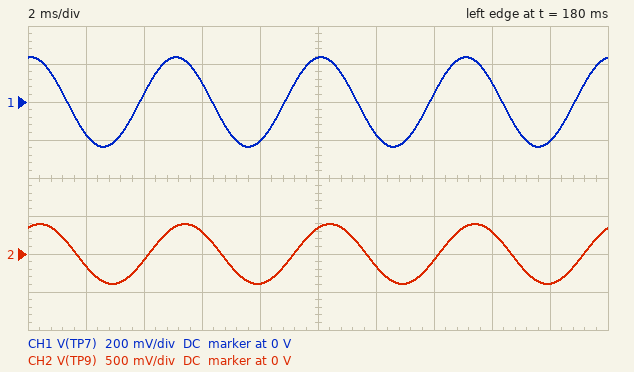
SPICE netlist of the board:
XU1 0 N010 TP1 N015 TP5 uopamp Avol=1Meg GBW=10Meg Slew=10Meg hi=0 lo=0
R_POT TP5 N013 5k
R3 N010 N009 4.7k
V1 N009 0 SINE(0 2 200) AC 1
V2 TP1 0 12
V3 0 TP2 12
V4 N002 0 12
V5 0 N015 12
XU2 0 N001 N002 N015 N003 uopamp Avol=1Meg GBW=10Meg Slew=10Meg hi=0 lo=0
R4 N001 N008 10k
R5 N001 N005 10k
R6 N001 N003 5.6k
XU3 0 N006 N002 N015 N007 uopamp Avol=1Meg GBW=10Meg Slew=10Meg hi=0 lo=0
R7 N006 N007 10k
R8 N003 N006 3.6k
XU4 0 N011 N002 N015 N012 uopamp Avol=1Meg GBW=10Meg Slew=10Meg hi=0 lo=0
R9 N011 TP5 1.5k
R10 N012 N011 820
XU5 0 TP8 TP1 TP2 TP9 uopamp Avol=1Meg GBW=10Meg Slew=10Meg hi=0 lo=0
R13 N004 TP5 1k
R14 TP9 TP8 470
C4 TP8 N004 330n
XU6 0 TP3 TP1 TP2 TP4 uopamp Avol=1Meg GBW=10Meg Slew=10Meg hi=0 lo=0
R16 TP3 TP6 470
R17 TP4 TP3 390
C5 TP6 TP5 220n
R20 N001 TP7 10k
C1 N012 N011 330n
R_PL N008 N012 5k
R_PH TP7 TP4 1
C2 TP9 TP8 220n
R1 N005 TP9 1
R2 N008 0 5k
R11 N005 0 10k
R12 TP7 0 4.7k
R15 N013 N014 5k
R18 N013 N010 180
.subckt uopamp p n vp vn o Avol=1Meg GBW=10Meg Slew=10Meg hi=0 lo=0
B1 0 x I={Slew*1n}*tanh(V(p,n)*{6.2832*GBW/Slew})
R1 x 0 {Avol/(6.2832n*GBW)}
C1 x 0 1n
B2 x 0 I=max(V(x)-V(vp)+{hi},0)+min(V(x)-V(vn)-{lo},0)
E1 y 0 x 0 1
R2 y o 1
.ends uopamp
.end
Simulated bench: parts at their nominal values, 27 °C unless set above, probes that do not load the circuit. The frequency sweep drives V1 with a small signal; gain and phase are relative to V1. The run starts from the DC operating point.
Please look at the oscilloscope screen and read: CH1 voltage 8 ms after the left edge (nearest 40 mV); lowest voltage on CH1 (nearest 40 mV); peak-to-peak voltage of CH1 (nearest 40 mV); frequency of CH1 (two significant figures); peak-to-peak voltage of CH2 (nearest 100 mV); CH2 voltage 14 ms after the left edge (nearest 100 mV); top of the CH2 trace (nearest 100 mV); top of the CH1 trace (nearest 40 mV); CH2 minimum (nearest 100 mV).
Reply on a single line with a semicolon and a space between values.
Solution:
-200 mV; -240 mV; 480 mV; 200 Hz; 800 mV; -100 mV; 400 mV; 240 mV; -400 mV
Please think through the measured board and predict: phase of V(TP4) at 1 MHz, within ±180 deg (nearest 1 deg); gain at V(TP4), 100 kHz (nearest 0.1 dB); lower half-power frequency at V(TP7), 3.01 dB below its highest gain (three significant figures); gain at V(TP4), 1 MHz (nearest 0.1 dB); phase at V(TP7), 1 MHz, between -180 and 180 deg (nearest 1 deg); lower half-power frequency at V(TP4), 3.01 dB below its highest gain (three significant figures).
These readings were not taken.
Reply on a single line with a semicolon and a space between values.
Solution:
-22 deg; -0.8 dB; 1.54 kHz; -1.1 dB; -22 deg; 1.54 kHz
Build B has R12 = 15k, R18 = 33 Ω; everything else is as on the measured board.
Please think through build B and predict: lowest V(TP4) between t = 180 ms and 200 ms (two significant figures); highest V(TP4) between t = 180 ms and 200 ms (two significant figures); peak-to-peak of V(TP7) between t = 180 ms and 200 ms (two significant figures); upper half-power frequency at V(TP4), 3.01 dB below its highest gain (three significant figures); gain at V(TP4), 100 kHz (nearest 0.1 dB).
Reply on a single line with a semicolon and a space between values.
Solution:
-230 mV; 230 mV; 460 mV; 3.29 MHz; -1.0 dB
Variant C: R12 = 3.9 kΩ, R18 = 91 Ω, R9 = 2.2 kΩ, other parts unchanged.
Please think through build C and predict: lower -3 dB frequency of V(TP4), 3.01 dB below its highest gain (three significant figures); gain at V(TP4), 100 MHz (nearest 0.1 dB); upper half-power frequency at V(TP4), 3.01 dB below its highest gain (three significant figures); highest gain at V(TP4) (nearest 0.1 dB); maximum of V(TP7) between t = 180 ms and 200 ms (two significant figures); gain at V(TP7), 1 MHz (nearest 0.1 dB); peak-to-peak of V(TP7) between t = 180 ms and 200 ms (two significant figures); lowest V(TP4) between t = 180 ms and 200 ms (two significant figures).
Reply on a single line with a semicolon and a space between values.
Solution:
1.54 kHz; -52.6 dB; 3.28 MHz; -0.9 dB; 230 mV; -1.3 dB; 460 mV; -230 mV
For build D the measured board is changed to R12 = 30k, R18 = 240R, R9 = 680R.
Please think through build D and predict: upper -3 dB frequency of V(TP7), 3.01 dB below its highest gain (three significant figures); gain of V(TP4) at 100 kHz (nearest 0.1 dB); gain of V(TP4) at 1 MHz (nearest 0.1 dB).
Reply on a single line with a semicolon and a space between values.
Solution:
3.25 MHz; -0.7 dB; -1.0 dB
